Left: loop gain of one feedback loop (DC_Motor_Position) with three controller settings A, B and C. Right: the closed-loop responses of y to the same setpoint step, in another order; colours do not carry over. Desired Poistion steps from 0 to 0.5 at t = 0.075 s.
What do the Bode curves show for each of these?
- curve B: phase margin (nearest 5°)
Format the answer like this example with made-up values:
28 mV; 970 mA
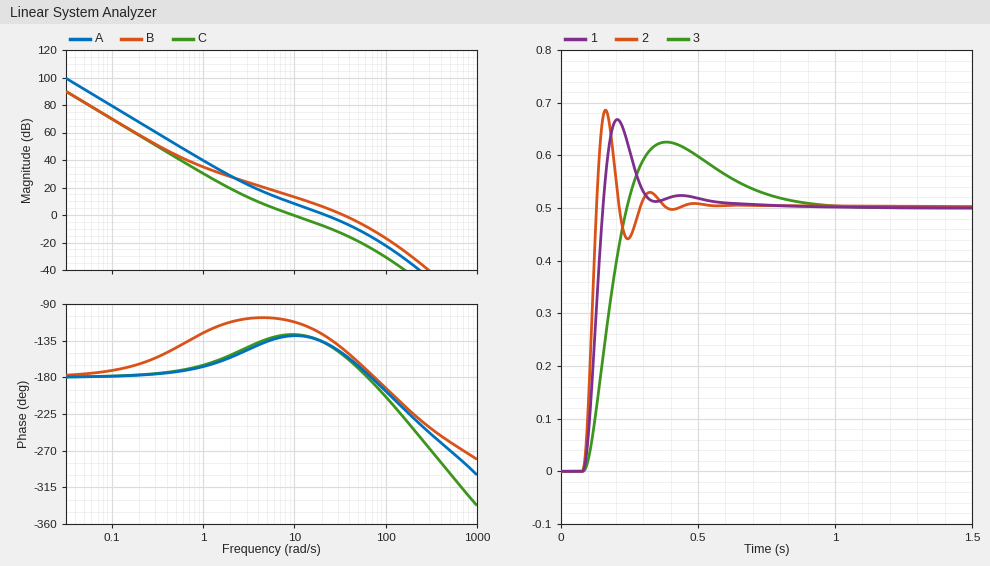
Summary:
35°
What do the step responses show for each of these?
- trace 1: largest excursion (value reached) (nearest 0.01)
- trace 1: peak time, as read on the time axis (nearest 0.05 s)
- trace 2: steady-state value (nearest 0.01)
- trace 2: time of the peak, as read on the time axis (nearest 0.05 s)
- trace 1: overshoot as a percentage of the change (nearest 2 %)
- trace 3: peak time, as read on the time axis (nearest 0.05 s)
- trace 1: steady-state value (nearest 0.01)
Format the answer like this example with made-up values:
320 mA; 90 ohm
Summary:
0.67; 0.20 s; 0.50; 0.15 s; 34 %; 0.40 s; 0.50
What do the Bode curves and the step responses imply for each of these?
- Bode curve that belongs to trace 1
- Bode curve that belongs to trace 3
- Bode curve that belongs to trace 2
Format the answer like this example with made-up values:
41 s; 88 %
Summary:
A; C; B
